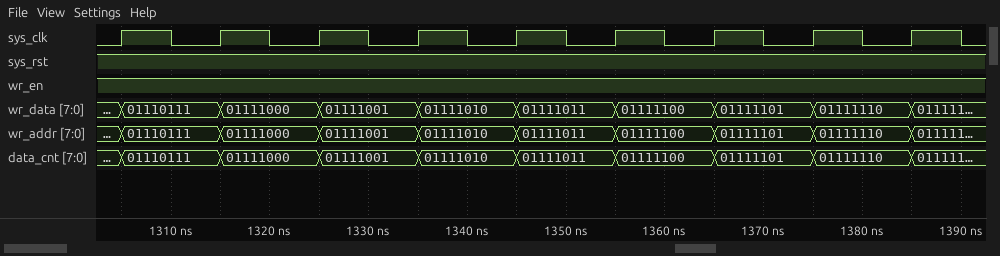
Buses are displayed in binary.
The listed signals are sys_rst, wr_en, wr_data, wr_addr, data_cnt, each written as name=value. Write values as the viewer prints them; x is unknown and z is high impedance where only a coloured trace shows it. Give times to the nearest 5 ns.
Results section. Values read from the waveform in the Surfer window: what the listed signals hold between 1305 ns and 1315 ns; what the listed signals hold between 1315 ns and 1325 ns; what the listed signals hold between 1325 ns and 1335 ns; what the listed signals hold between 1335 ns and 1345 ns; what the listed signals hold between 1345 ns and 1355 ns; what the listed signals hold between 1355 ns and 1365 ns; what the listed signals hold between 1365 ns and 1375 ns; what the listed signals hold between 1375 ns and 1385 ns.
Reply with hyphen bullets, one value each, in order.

- sys_rst=1, wr_en=1, wr_data=01110111, wr_addr=01110111, data_cnt=01110111
- sys_rst=1, wr_en=1, wr_data=01111000, wr_addr=01111000, data_cnt=01111000
- sys_rst=1, wr_en=1, wr_data=01111001, wr_addr=01111001, data_cnt=01111001
- sys_rst=1, wr_en=1, wr_data=01111010, wr_addr=01111010, data_cnt=01111010
- sys_rst=1, wr_en=1, wr_data=01111011, wr_addr=01111011, data_cnt=01111011
- sys_rst=1, wr_en=1, wr_data=01111100, wr_addr=01111100, data_cnt=01111100
- sys_rst=1, wr_en=1, wr_data=01111101, wr_addr=01111101, data_cnt=01111101
- sys_rst=1, wr_en=1, wr_data=01111110, wr_addr=01111110, data_cnt=01111110
